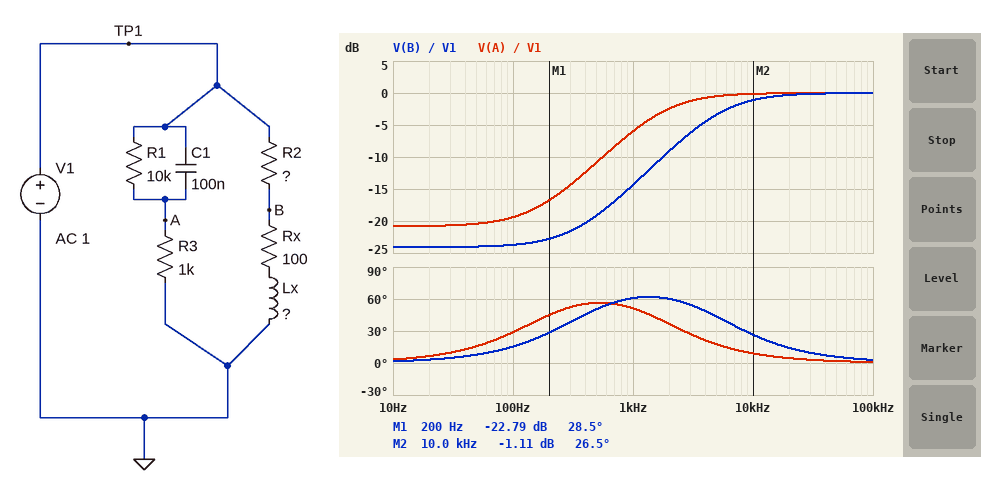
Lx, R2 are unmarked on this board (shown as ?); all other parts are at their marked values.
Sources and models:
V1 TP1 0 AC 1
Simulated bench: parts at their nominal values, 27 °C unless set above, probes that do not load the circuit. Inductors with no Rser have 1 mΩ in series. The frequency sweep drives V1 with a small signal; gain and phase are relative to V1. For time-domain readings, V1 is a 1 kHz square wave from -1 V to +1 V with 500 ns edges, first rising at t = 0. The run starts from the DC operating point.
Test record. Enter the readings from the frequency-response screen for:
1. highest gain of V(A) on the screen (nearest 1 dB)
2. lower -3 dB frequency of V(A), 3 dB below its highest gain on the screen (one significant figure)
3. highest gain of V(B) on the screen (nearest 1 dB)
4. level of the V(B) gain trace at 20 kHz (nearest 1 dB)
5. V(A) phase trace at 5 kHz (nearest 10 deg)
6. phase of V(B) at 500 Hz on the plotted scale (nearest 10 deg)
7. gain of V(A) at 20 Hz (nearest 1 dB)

0 dB
2 kHz
0 dB
0 dB
20 deg
50 deg
-21 dB
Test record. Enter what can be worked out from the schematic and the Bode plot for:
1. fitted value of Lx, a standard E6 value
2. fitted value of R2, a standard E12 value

47 mH
1.5 kΩ
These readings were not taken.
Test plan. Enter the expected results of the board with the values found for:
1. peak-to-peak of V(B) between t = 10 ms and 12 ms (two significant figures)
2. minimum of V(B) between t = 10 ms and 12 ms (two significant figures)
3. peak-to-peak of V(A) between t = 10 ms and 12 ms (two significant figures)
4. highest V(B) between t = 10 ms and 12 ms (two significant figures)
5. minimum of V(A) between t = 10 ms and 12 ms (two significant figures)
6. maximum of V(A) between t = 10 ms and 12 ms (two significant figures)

3.8 V
-1.9 V
3.8 V
1.9 V
-1.9 V
1.9 V
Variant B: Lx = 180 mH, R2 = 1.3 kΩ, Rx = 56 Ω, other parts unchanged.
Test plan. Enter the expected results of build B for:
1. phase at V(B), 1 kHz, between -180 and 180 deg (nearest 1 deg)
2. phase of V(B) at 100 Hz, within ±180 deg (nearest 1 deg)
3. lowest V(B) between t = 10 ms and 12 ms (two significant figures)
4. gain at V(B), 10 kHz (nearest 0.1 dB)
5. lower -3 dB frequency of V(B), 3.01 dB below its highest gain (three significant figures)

47 deg
59 deg
-1.9 V
-0.1 dB
1.20 kHz
